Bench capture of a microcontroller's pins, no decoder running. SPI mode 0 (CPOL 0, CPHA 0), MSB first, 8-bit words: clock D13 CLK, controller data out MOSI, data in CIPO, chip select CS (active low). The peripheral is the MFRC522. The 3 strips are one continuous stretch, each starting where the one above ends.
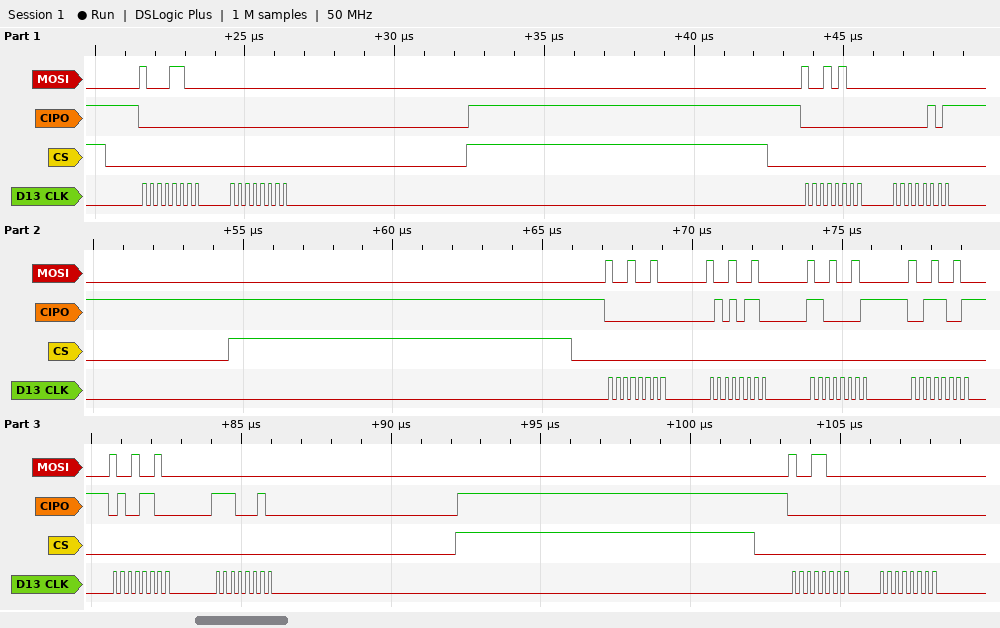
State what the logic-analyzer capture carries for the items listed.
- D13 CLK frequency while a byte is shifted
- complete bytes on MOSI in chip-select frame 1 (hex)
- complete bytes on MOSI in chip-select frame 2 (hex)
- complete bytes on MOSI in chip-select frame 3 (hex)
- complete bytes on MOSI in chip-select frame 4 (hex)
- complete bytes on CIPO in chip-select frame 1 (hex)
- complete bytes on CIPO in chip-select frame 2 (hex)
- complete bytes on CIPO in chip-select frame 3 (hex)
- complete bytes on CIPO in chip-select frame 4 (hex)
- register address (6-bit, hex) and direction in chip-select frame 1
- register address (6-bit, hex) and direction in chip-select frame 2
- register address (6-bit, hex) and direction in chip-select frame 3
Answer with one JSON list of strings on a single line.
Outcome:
["4 MHz", "8C 00", "94 00", "92 92 92 92 92 00", "98 00", "00 00", "00 05", "00 56 C1 39 4C E2", "00 00", "0x06 read", "0x0A read", "0x09 read"]
